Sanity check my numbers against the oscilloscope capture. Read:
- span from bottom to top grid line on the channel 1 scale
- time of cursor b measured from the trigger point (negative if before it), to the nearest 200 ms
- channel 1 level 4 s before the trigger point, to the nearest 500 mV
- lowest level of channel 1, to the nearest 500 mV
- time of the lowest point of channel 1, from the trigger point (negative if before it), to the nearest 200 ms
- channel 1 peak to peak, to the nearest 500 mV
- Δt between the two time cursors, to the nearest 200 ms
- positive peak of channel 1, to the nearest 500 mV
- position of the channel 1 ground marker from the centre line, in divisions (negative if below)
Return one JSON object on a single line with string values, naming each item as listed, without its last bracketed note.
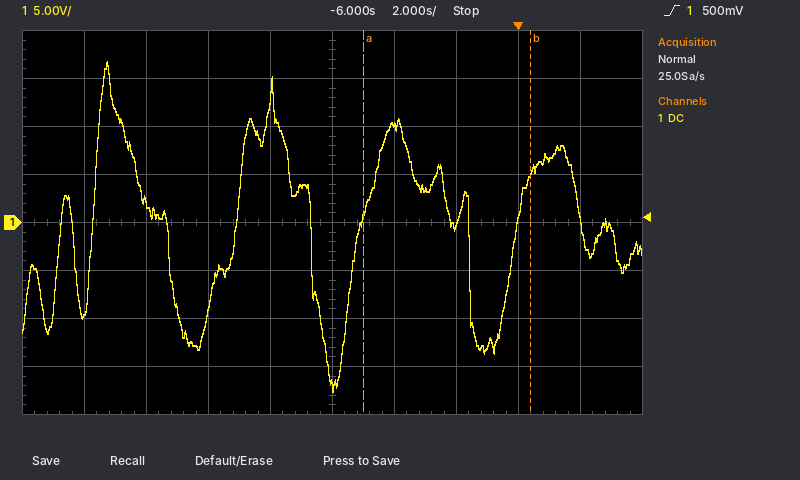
{"span from bottom to top grid line on the channel 1 scale": "40 V", "time of cursor b measured from the trigger point (negative if before it), to the nearest 200 ms": "+400 ms", "channel 1 level 4 s before the trigger point, to the nearest 500 mV": "10.0 V", "lowest level of channel 1, to the nearest 500 mV": "-17.5 V", "time of the lowest point of channel 1, from the trigger point (negative if before it), to the nearest 200 ms": "-6.0 s", "channel 1 peak to peak, to the nearest 500 mV": "34.5 V", "Δt between the two time cursors, to the nearest 200 ms": "5.4 s", "positive peak of channel 1, to the nearest 500 mV": "17.0 V", "position of the channel 1 ground marker from the centre line, in divisions": "0.0 div"}
